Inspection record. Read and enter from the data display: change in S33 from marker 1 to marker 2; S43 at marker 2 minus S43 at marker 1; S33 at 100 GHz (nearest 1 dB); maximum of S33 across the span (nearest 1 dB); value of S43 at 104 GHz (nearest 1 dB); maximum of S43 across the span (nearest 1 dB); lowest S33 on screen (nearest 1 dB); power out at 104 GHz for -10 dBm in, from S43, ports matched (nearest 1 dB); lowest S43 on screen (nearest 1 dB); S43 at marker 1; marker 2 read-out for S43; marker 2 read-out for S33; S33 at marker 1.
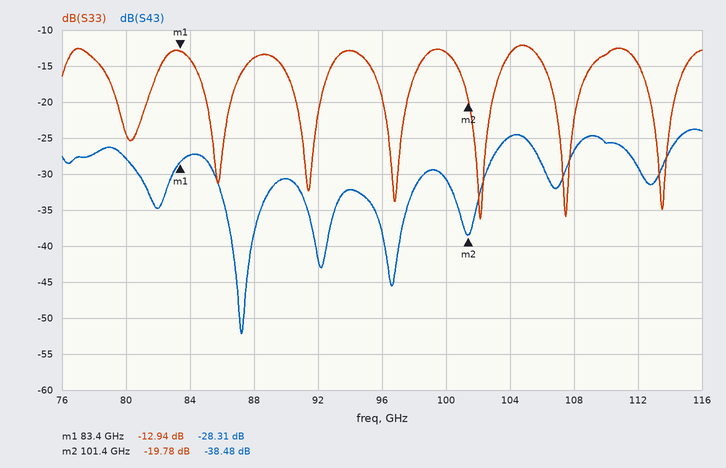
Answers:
-6.84 dB
-10.17 dB
-13 dB
-12 dB
-25 dB
-24 dB
-36 dB
-35 dBm
-52 dB
-28.31 dB
-38.48 dB
-19.78 dB
-12.94 dB
